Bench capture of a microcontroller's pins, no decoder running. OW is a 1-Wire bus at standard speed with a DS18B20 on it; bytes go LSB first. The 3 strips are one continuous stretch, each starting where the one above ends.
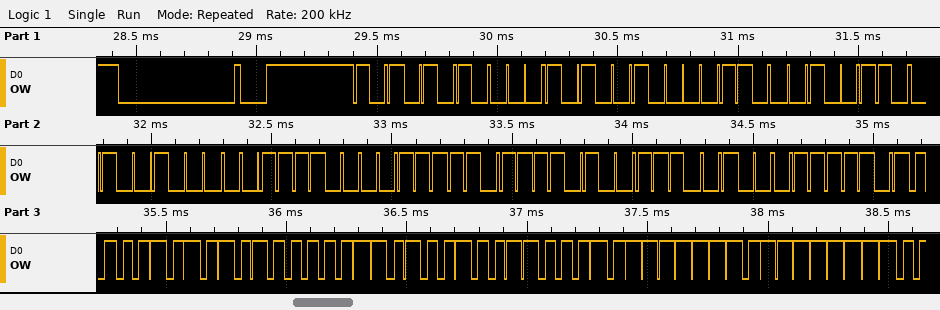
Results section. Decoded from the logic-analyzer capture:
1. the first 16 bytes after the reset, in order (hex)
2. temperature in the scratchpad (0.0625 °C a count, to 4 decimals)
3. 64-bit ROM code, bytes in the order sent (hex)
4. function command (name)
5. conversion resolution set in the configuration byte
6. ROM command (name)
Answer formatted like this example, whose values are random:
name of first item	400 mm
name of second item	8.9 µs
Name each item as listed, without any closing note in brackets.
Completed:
the first 16 bytes after the reset, in order	55 28 61 64 12 3C 7C 2F 27 BE 50 05 4B 46 7F FF
temperature in the scratchpad	85.0000 °C
64-bit ROM code, bytes in the order sent	28 61 64 12 3C 7C 2F 27
function command	Read Scratchpad
conversion resolution set in the configuration byte	12 bits
ROM command	Match ROM
